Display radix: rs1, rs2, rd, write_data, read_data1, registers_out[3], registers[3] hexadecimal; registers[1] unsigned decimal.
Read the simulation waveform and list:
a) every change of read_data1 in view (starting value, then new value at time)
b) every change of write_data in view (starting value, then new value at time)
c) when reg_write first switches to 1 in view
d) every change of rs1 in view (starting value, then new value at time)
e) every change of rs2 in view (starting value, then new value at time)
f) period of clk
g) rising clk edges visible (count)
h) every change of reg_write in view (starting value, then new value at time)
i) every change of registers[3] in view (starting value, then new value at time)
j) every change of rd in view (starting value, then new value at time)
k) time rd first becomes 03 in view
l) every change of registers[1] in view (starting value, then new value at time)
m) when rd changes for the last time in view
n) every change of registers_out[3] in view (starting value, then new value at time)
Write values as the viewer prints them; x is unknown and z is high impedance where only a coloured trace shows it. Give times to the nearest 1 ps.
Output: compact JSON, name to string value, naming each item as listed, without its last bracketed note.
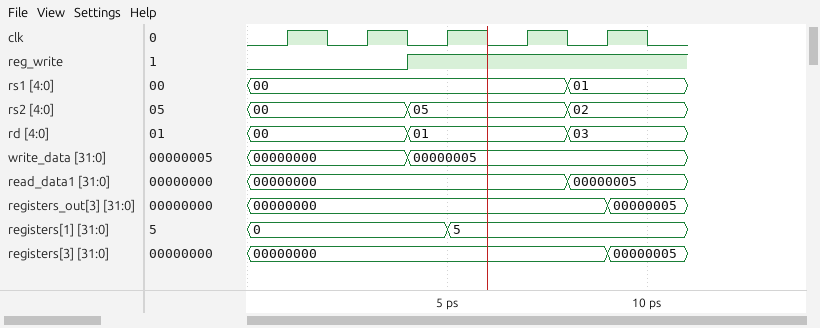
{"every change of read_data1 in view": "00000000, 00000005 at 8 ps", "every change of write_data in view": "00000000, 00000005 at 4 ps", "when reg_write first switches to 1 in view": "4 ps", "every change of rs1 in view": "00, 01 at 8 ps", "every change of rs2 in view": "00, 05 at 4 ps, 02 at 8 ps", "period of clk": "2 ps", "rising clk edges visible": "5", "every change of reg_write in view": "0, 1 at 4 ps", "every change of registers[3] in view": "00000000, 00000005 at 9 ps", "every change of rd in view": "00, 01 at 4 ps, 03 at 8 ps", "time rd first becomes 03 in view": "8 ps", "every change of registers[1] in view": "0, 5 at 5 ps", "when rd changes for the last time in view": "8 ps", "every change of registers_out[3] in view": "00000000, 00000005 at 9 ps"}
